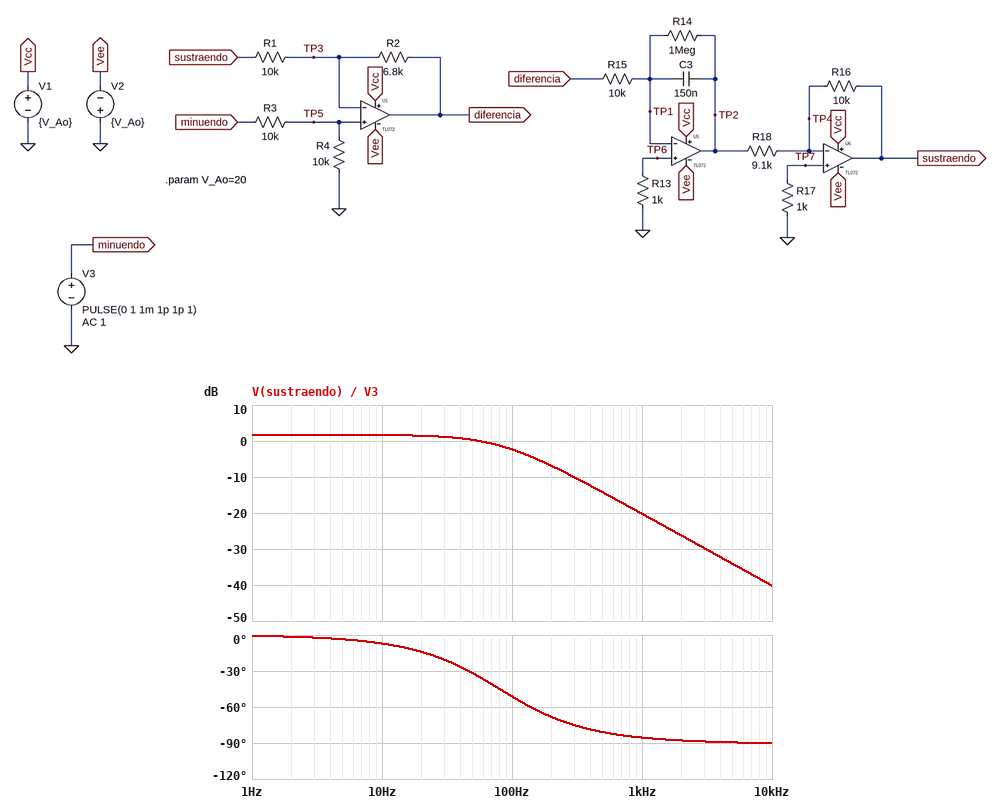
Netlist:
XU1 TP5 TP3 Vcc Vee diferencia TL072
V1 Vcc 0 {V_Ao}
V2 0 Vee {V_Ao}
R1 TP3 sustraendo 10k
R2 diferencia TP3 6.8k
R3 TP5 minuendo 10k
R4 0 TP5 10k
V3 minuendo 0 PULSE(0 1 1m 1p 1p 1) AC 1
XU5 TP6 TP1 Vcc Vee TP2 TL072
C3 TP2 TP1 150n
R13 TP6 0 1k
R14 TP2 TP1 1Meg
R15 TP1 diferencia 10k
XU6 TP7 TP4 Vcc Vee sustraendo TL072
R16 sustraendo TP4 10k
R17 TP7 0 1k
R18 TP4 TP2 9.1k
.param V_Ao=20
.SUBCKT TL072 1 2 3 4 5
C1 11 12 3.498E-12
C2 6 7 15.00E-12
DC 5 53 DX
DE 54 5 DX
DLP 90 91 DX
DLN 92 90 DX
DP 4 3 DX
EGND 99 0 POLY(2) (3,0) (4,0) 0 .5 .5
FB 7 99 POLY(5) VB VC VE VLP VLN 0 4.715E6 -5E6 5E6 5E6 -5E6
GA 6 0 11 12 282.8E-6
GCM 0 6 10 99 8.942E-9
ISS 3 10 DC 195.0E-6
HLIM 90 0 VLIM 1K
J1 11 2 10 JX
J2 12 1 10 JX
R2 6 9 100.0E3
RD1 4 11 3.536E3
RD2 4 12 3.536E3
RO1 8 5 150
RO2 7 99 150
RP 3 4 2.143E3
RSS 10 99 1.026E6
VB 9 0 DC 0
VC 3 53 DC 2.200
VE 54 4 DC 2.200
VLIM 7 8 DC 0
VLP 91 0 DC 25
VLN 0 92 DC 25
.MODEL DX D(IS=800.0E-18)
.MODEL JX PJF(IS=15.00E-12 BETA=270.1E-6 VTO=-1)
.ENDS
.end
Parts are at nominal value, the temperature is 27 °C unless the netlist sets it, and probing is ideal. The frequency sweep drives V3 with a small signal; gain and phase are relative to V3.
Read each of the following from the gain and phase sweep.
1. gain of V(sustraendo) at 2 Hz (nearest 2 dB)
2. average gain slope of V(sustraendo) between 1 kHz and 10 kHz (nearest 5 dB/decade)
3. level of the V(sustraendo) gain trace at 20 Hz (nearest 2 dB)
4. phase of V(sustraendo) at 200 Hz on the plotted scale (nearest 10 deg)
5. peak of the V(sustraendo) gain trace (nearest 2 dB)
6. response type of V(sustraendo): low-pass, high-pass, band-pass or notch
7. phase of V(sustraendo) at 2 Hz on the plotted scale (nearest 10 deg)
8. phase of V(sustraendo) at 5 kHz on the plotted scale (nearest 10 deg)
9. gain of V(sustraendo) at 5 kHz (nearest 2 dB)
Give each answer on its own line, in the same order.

2 dB
-20 dB/decade
2 dB
-70 deg
2 dB
low-pass
0 deg
-90 deg
-34 dB
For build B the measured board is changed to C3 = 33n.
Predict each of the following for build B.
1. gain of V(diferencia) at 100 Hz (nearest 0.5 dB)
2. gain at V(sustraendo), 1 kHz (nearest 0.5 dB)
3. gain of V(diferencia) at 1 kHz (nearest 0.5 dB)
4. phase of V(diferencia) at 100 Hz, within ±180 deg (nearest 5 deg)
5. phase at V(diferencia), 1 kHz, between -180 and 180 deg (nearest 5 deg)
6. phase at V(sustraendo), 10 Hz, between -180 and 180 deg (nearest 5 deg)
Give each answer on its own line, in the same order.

-13.0 dB
-7.5 dB
-2.0 dB
70 deg
20 deg
0 deg
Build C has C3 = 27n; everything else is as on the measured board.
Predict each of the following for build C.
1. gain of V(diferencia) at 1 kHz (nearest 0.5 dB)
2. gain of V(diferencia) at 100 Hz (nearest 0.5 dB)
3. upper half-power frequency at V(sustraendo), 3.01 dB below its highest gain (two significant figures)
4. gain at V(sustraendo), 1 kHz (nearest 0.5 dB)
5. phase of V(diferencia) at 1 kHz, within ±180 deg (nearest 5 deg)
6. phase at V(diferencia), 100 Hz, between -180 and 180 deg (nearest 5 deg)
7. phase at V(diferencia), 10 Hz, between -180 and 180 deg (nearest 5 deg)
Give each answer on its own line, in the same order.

-2.5 dB
-14.5 dB
450 Hz
-6.0 dB
25 deg
75 deg
60 deg
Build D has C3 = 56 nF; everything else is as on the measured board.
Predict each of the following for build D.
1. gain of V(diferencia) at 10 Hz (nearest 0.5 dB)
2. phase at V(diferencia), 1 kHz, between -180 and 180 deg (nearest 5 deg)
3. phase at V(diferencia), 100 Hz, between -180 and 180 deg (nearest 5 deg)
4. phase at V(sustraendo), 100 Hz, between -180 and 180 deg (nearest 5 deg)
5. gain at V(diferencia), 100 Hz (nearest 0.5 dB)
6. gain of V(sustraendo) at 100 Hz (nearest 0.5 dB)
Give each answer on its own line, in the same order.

-28.0 dB
10 deg
65 deg
-25 deg
-9.0 dB
1.0 dB
